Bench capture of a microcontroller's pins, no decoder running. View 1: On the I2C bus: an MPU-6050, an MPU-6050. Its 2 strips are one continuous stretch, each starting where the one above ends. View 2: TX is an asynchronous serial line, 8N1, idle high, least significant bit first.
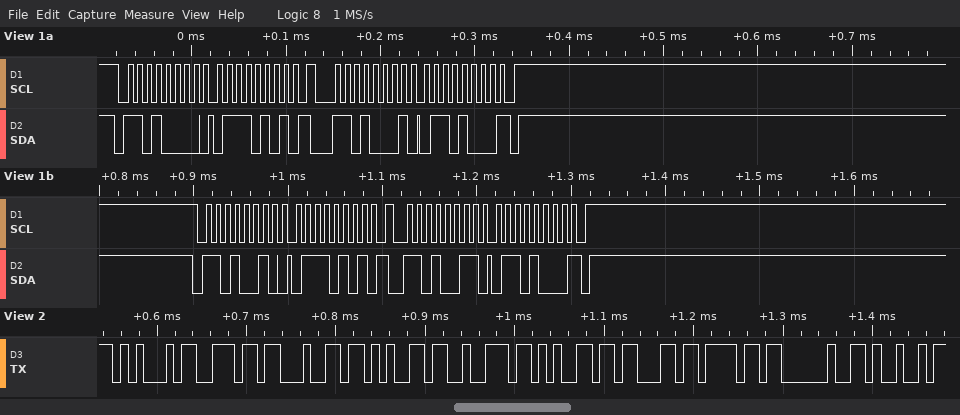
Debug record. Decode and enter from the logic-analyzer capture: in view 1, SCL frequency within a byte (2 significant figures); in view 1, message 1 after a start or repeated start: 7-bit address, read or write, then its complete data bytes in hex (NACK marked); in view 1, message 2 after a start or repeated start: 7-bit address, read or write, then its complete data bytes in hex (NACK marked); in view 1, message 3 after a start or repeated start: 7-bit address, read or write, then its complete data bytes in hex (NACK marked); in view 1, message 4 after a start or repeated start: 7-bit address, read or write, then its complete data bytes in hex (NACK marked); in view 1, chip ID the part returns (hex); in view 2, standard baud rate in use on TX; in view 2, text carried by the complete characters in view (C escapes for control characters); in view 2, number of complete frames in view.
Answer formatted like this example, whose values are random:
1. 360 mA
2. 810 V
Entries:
1. 100 kHz
2. 0x68 write: 75
3. 0x68 read: 68 NACK
4. 0x69 write: 75
5. 0x69 read: 68 NACK
6. 0x68
7. 115200 baud
8. "Endereco I"
9. 10
